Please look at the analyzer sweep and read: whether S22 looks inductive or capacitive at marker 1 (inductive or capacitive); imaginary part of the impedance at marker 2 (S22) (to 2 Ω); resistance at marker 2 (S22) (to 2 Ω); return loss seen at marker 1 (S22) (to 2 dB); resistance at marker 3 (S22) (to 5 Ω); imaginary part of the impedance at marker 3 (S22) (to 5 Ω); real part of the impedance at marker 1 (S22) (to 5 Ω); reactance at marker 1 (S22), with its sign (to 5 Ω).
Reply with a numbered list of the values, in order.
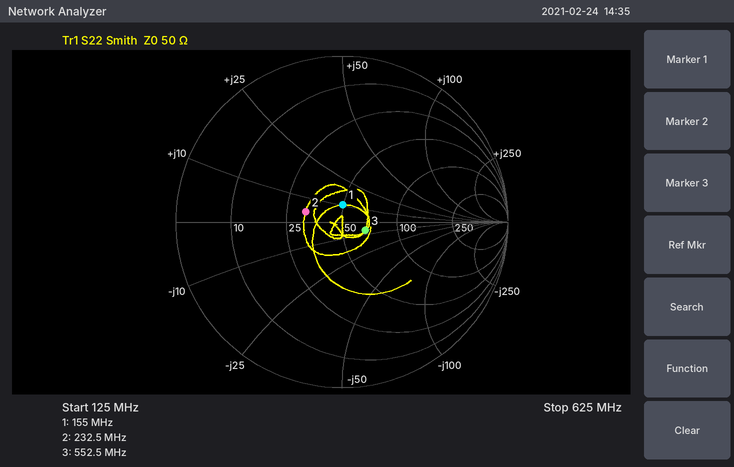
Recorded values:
1. inductive
2. +4 Ω
3. 32 Ω
4. 20 dB
5. 65 Ω
6. -5 Ω
7. 50 Ω
8. +10 Ω
